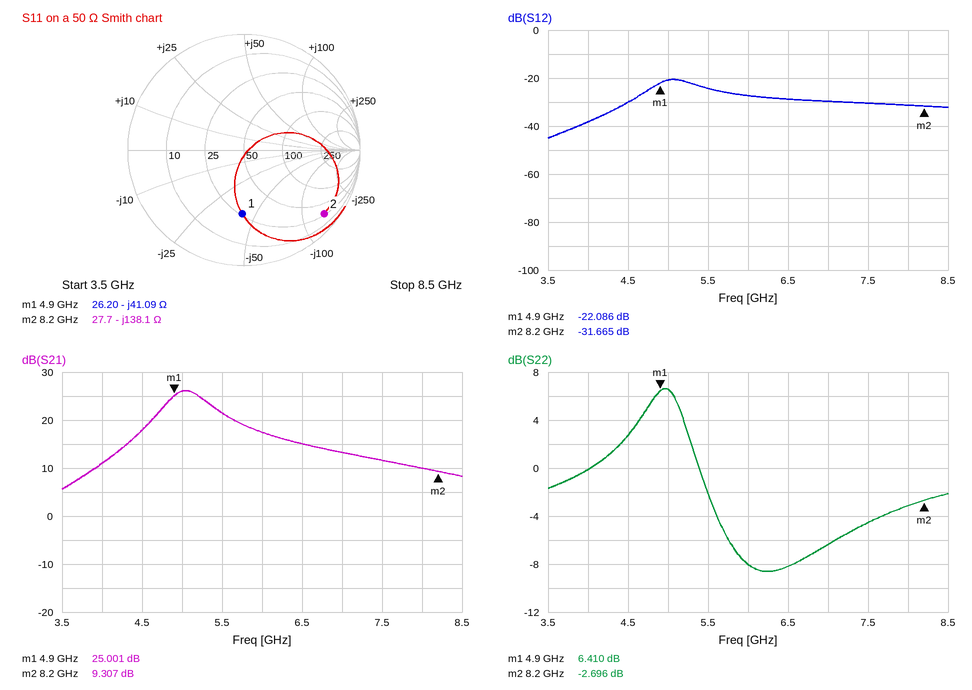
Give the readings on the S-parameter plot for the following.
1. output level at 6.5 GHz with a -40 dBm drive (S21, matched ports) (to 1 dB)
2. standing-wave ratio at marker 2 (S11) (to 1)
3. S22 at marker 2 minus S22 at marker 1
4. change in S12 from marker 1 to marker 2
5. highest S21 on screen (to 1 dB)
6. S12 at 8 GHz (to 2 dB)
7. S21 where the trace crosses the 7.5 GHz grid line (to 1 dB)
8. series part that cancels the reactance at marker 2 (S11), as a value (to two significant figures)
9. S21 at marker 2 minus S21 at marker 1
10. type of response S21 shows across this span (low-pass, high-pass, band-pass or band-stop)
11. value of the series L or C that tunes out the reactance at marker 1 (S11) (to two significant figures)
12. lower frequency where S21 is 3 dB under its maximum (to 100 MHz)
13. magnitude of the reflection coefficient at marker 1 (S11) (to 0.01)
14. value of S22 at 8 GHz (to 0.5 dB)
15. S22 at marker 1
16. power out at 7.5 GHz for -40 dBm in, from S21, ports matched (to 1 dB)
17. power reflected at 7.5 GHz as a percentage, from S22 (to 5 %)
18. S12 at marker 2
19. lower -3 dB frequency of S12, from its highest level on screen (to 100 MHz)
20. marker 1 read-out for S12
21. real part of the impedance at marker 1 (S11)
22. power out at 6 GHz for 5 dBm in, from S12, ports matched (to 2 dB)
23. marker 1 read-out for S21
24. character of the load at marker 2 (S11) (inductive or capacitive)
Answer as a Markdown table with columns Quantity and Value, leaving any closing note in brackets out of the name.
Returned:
| Quantity | Value |
|---|---|
| output level at 6.5 GHz with a -40 dBm drive (S21, matched ports) | -25 dBm |
| standing-wave ratio at marker 2 (S11) | 16 |
| S22 at marker 2 minus S22 at marker 1 | -9.106 dB |
| change in S12 from marker 1 to marker 2 | -9.579 dB |
| highest S21 on screen | 26 dB |
| S12 at 8 GHz | -32 dB |
| S21 where the trace crosses the 7.5 GHz grid line | 12 dB |
| series part that cancels the reactance at marker 2 (S11), as a value | 2.7 nH |
| S21 at marker 2 minus S21 at marker 1 | -15.694 dB |
| type of response S21 shows across this span | band-pass |
| value of the series L or C that tunes out the reactance at marker 1 (S11) | 1.3 nH |
| lower frequency where S21 is 3 dB under its maximum | 4.8 GHz |
| magnitude of the reflection coefficient at marker 1 (S11) | 0.55 |
| value of S22 at 8 GHz | -3.0 dB |
| S22 at marker 1 | 6.410 dB |
| power out at 7.5 GHz for -40 dBm in, from S21, ports matched | -28 dBm |
| power reflected at 7.5 GHz as a percentage, from S22 | 35 % |
| S12 at marker 2 | -31.665 dB |
| lower -3 dB frequency of S12, from its highest level on screen | 4.8 GHz |
| marker 1 read-out for S12 | -22.086 dB |
| real part of the impedance at marker 1 | 26.20 Ω |
| power out at 6 GHz for 5 dBm in, from S12, ports matched | -22 dBm |
| marker 1 read-out for S21 | 25.001 dB |
| character of the load at marker 2 (S11) | capacitive |
